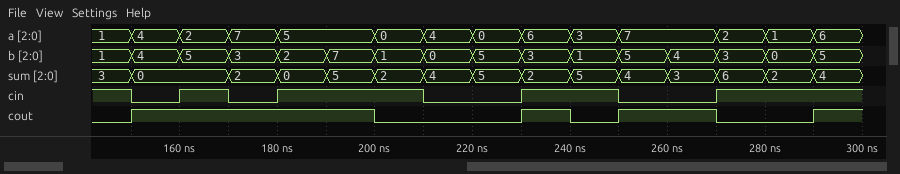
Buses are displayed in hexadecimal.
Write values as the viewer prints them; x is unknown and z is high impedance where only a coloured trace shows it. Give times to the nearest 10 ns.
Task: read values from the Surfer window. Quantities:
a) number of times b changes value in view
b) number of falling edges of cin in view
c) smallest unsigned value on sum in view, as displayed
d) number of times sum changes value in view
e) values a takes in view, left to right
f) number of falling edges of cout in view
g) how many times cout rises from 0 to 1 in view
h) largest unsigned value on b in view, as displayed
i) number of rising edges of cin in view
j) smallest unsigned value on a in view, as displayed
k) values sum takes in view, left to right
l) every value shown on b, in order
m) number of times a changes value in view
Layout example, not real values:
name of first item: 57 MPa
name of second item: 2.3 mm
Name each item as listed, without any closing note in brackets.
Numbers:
number of times b changes value in view: 15
number of falling edges of cin in view: 4
smallest unsigned value on sum in view, as displayed: 0
number of times sum changes value in view: 14
values a takes in view, left to right: 1, 4, 2, 7, 5, 0, 4, 0, 6, 3, 7, 2, 1, 6
number of falling edges of cout in view: 3
how many times cout rises from 0 to 1 in view: 4
largest unsigned value on b in view, as displayed: 7
number of rising edges of cin in view: 4
smallest unsigned value on a in view, as displayed: 0
values sum takes in view, left to right: 3, 0, 2, 0, 5, 2, 4, 5, 2, 5, 4, 3, 6, 2, 4
every value shown on b, in order: 1, 4, 5, 3, 2, 7, 1, 0, 5, 3, 1, 5, 4, 3, 0, 5
number of times a changes value in view: 13
